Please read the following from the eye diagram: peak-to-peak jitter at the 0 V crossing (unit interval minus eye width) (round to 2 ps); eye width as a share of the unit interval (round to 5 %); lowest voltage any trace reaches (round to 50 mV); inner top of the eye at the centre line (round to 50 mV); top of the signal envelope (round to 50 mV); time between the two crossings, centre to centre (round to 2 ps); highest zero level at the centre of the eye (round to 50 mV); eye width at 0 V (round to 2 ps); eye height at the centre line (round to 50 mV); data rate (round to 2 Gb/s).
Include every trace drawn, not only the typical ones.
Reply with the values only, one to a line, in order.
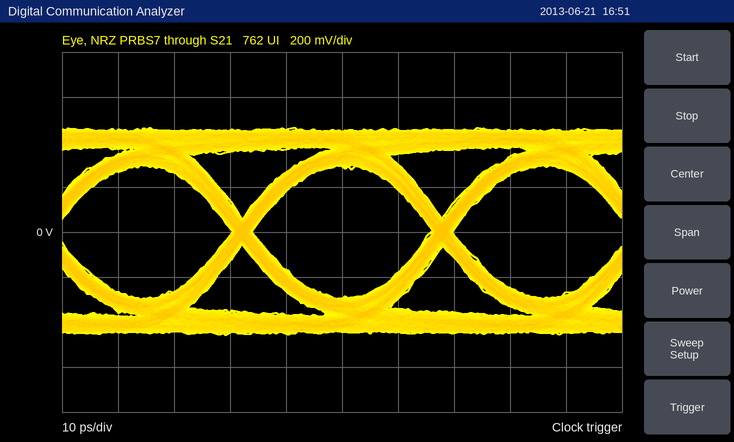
4 ps
90 %
-450 mV
300 mV
450 mV
36 ps
-300 mV
32 ps
600 mV
28 Gb/s
